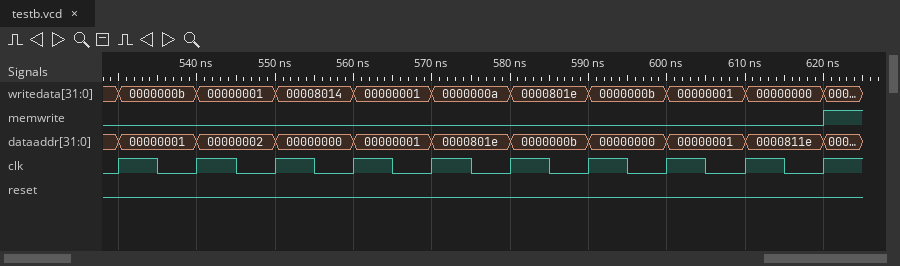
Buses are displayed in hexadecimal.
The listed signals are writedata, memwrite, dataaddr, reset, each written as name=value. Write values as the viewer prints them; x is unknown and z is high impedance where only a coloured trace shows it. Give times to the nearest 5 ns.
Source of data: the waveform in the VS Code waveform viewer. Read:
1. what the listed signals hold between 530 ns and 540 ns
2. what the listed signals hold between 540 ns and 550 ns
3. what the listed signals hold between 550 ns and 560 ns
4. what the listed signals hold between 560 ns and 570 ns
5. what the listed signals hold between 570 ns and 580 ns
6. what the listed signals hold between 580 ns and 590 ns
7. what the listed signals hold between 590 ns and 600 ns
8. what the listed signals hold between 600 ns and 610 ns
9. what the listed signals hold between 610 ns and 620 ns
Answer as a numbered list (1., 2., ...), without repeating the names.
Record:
1. writedata=0000000b, memwrite=0, dataaddr=00000001, reset=0
2. writedata=00000001, memwrite=0, dataaddr=00000002, reset=0
3. writedata=00008014, memwrite=0, dataaddr=00000000, reset=0
4. writedata=00000001, memwrite=0, dataaddr=00000001, reset=0
5. writedata=0000000a, memwrite=0, dataaddr=0000801e, reset=0
6. writedata=0000801e, memwrite=0, dataaddr=0000000b, reset=0
7. writedata=0000000b, memwrite=0, dataaddr=00000000, reset=0
8. writedata=00000001, memwrite=0, dataaddr=00000001, reset=0
9. writedata=00000000, memwrite=0, dataaddr=0000811e, reset=0
